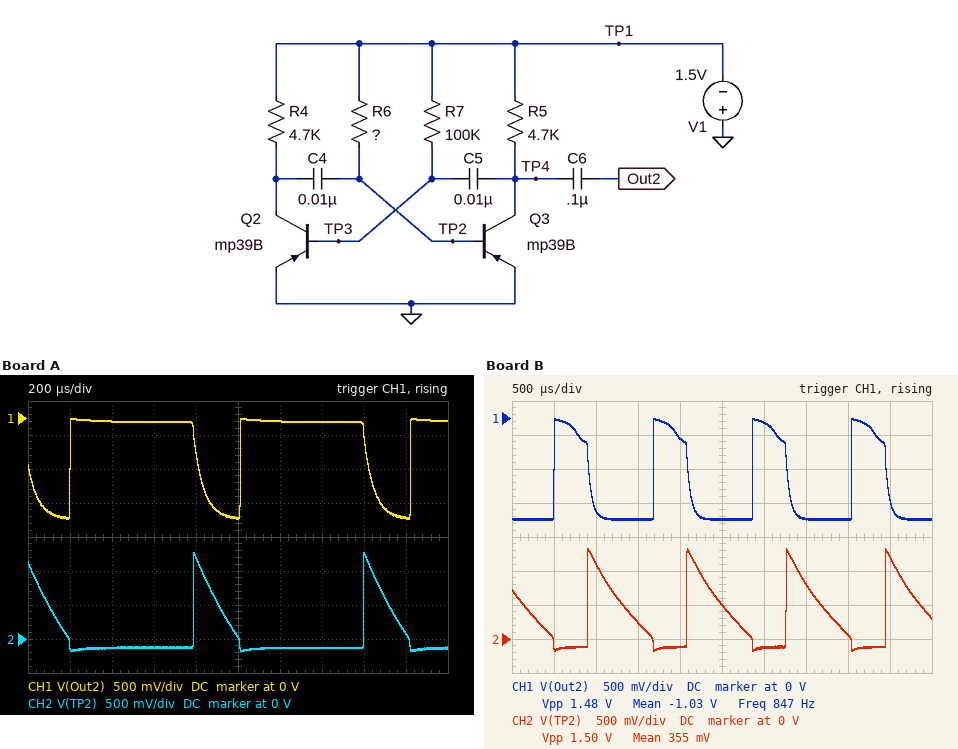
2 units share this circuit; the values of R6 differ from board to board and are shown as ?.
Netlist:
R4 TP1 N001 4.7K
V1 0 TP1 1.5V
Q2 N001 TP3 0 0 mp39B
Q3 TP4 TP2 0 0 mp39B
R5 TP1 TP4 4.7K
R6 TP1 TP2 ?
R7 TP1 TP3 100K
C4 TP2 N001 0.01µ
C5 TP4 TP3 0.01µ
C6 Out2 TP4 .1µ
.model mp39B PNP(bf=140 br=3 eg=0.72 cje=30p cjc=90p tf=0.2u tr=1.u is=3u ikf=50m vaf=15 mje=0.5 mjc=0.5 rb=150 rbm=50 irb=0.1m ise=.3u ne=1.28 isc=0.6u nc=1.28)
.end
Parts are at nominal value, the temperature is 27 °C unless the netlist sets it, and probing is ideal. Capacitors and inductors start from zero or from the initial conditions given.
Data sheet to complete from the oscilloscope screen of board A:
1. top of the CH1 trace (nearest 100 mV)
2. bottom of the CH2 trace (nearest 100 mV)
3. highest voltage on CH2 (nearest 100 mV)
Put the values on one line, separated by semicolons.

0 V; -200 mV; 1.3 V
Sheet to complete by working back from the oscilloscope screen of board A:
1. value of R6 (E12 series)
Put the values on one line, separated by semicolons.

39 kΩ
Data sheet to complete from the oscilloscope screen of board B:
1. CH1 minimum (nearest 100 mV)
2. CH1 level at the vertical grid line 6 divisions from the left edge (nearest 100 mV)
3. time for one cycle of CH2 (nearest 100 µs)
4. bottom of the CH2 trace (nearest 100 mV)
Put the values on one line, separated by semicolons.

-1.5 V; -100 mV; 1.2 ms; -200 mV
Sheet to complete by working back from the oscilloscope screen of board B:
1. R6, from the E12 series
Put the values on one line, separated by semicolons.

150 kΩ
